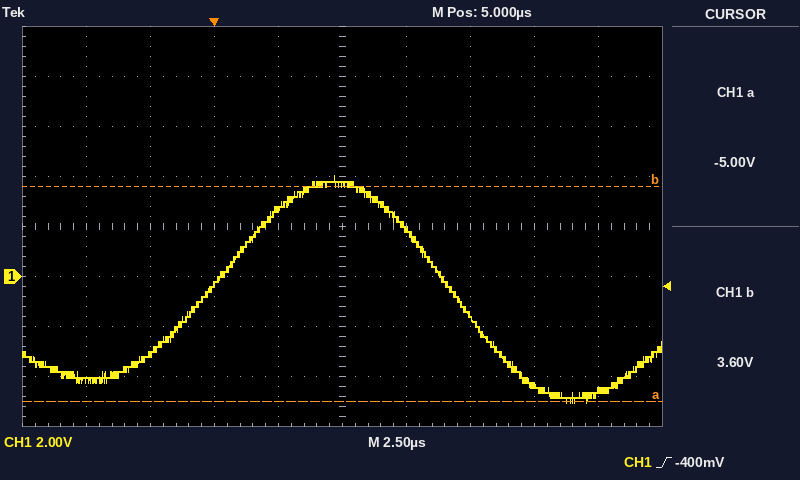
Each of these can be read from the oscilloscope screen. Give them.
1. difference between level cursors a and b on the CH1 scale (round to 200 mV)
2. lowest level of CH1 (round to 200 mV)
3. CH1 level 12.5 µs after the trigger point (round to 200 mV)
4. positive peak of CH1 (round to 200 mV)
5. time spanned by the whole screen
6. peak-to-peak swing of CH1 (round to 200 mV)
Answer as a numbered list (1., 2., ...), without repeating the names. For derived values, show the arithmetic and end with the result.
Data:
1. 8.6 V
2. -5.0 V
3. -4.4 V
4. 4.0 V
5. 25 µs
6. 4.0 V − (-5.0 V) = 9.0 V
